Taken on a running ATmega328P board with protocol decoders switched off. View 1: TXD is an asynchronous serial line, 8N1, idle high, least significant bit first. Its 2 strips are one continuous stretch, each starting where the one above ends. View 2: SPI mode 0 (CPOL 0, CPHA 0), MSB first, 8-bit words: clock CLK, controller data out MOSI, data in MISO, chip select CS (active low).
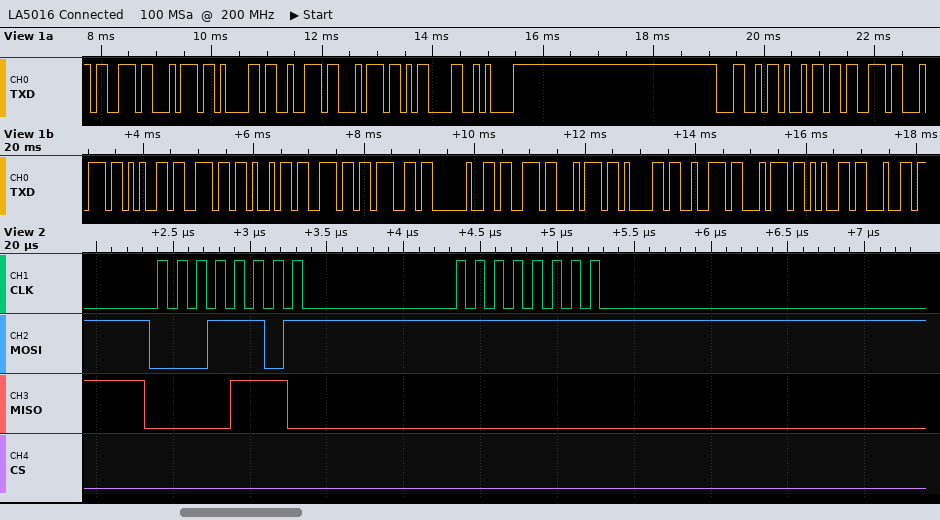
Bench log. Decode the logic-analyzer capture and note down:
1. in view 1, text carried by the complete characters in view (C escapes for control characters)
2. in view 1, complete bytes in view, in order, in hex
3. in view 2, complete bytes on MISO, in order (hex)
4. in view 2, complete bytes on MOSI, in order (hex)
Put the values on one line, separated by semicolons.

"start\r\nListening started"; 73 74 61 72 74 0D 0A 4C 69 73 74 65 6E 69 6E 67 20 73 74 61 72 74 65 64; 0E 00; 1D FF
